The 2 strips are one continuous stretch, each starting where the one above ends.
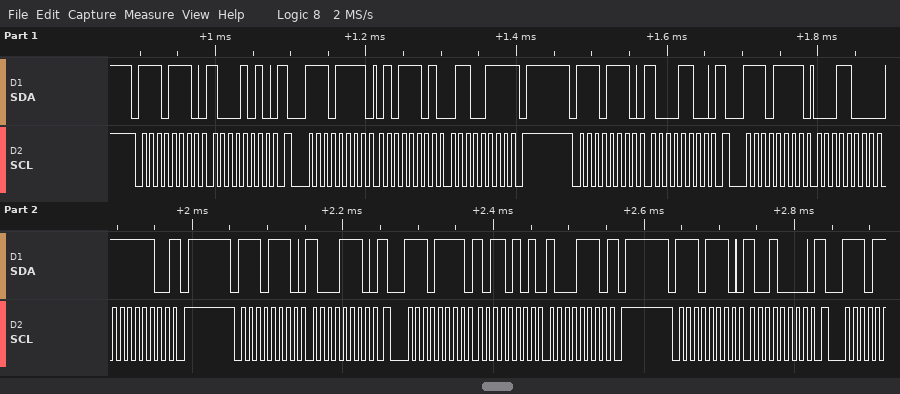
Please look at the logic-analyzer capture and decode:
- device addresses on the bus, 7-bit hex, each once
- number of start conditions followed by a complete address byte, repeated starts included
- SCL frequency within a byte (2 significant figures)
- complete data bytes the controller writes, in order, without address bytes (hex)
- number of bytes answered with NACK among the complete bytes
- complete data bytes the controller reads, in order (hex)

0x77
7
100 kHz
8A 8C 8E 90
3
5D 67 18 FC B5 8E
